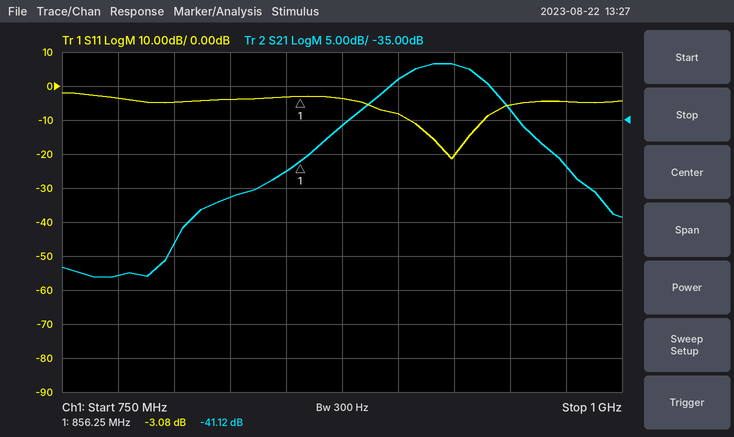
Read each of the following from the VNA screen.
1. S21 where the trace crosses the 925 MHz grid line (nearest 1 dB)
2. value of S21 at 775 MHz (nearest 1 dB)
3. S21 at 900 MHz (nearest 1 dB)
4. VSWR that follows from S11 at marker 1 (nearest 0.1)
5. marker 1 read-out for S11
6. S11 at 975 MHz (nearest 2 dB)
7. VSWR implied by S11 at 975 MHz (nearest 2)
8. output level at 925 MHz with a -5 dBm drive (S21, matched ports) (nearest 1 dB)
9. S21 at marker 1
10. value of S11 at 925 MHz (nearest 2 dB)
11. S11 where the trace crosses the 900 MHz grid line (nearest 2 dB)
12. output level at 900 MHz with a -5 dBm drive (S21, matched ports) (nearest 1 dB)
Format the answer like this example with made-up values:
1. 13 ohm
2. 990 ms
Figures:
1. -27 dB
2. -58 dB
3. -29 dB
4. 5.7
5. -3.08 dB
6. -4 dB
7. 4
8. -32 dBm
9. -41.12 dB
10. -20 dB
11. -8 dB
12. -34 dBm
